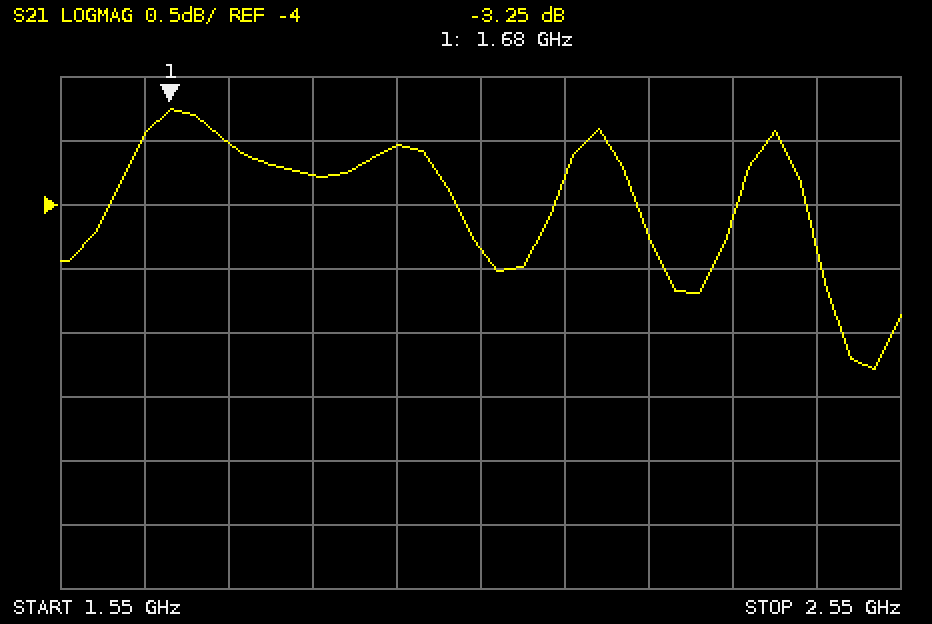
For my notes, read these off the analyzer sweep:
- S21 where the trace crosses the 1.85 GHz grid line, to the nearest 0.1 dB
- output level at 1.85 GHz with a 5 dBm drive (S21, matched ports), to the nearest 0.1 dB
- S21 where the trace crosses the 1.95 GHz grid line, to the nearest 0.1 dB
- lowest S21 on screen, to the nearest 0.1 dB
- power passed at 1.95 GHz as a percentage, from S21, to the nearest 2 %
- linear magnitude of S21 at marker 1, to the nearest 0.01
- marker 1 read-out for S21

-3.8 dB
1.2 dBm
-3.5 dB
-5.3 dB
44 %
0.69
-3.25 dB
